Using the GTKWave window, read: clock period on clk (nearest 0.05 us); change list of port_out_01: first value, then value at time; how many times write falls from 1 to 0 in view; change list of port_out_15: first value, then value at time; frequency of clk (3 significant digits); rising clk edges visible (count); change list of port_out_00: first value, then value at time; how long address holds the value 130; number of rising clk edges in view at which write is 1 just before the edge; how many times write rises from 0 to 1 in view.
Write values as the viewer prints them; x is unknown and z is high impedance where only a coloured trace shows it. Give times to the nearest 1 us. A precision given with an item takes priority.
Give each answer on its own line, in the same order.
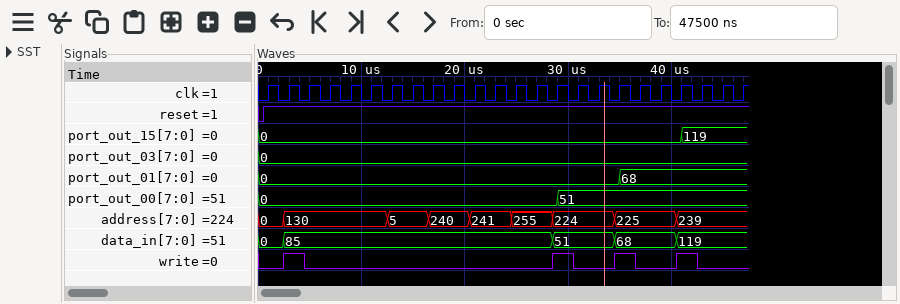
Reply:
2 us
0, 68 at 35 us
4
0, 119 at 41 us
500 kHz
24
0, 51 at 29 us
10 us
4
4
